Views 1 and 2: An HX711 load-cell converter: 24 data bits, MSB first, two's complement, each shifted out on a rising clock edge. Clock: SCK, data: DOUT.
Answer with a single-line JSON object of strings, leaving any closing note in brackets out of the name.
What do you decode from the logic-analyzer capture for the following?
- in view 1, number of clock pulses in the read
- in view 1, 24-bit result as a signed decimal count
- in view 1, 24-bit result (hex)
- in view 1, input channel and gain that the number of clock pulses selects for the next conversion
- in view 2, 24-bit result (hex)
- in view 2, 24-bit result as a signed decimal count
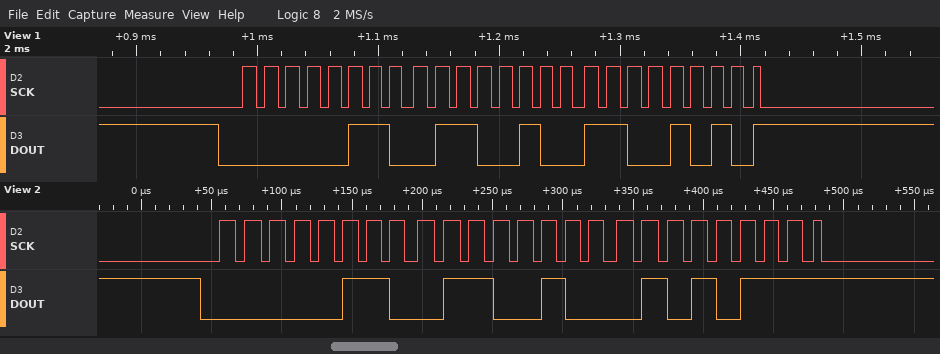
{"in view 1, number of clock pulses in the read": "25", "in view 1, 24-bit result as a signed decimal count": "419018", "in view 1, 24-bit result": "0x0664CA", "in view 1, input channel and gain that the number of clock pulses selects for the next conversion": "channel A, gain 128", "in view 2, 24-bit result": "0x066457", "in view 2, 24-bit result as a signed decimal count": "418903"}
